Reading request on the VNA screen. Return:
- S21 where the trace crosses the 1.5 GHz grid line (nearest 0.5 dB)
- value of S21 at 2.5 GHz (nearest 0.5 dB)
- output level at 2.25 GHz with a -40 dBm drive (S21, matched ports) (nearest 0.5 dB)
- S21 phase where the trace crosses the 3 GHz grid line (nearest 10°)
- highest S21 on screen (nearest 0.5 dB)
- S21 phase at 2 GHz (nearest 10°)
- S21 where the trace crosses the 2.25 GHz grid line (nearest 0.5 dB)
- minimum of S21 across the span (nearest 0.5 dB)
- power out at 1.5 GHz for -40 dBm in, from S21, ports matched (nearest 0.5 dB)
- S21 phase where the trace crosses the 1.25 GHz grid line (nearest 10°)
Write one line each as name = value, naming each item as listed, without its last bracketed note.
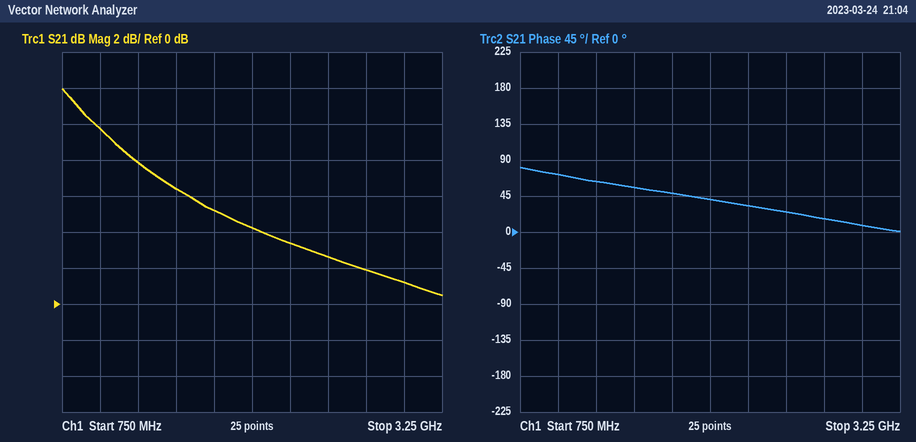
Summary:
S21 where the trace crosses the 1.5 GHz grid line = 6.5 dB
value of S21 at 2.5 GHz = 2.5 dB
output level at 2.25 GHz with a -40 dBm drive (S21, matched ports) = -36.5 dBm
S21 phase where the trace crosses the 3 GHz grid line = 10°
highest S21 on screen = 12.0 dB
S21 phase at 2 GHz = 40°
S21 where the trace crosses the 2.25 GHz grid line = 3.5 dB
minimum of S21 across the span = 0.5 dB
power out at 1.5 GHz for -40 dBm in, from S21, ports matched = -33.5 dBm
S21 phase where the trace crosses the 1.25 GHz grid line = 60°
